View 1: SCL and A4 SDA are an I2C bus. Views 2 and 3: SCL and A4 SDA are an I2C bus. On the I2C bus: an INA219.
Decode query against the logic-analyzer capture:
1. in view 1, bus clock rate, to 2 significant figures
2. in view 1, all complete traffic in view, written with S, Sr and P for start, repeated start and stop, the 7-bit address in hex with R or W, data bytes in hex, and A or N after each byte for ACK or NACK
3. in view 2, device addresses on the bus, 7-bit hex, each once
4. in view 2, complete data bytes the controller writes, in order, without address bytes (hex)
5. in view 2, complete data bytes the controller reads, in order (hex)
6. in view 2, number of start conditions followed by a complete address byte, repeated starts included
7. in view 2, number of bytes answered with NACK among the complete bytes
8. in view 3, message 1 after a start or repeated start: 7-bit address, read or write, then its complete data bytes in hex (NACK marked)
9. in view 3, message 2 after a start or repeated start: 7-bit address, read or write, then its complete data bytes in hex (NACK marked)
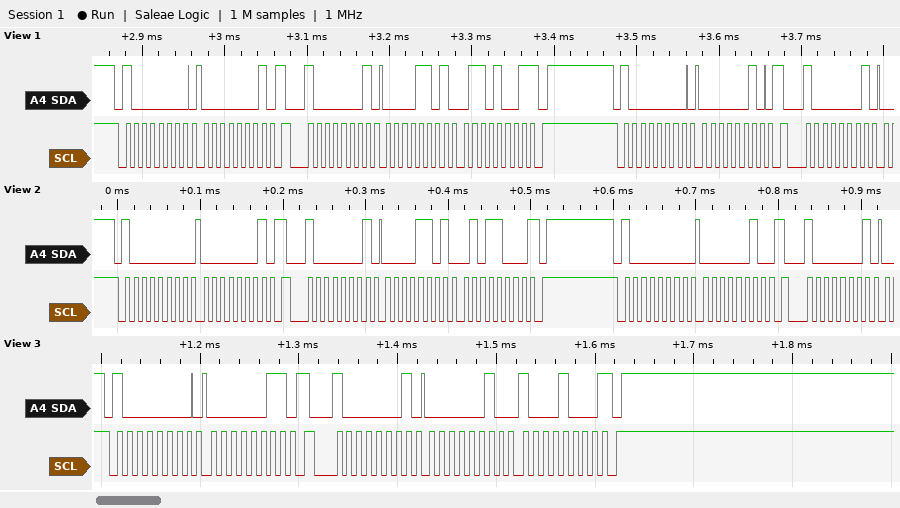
100 kHz
S 40W A 01 A Sr 40R A 0D A 69 N P S 40W A 02 A Sr 40R A
0x40
01 02
0D 58
4
1
0x40 write: 03
0x40 read: 02 88 NACK
